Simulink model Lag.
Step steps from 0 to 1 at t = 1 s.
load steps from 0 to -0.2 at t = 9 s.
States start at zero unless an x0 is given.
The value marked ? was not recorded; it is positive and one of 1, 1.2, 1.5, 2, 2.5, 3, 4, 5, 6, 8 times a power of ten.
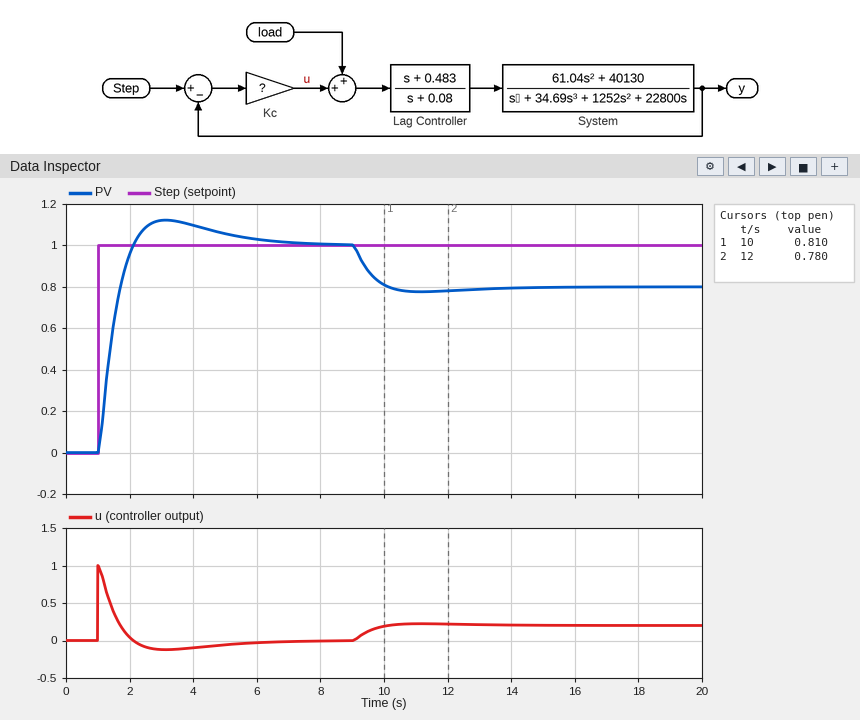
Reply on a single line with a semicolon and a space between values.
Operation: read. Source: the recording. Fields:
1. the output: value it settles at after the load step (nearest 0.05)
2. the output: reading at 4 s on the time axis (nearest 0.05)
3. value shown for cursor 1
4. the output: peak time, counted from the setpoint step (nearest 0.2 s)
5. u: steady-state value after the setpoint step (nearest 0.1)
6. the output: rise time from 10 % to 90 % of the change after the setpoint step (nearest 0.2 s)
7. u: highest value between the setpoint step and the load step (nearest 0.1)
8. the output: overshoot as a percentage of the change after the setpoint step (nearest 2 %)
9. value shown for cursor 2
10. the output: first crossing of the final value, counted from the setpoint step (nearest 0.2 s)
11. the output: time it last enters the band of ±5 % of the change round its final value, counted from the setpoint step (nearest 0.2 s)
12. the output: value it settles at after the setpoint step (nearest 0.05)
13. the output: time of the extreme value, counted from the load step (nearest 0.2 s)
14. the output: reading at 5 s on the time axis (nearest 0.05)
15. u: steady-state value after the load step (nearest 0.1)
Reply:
0.80; 1.10; 0.810; 2.2 s; 0.0; 0.8 s; 1.0; 12 %; 0.780; 1.2 s; 4.2 s; 1.00; 2.2 s; 1.05; 0.2
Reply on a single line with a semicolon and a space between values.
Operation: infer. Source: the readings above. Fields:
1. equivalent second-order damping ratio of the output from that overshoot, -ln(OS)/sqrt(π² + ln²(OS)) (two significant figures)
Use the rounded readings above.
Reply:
0.56
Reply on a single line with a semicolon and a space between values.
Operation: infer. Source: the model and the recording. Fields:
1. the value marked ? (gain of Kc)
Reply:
1
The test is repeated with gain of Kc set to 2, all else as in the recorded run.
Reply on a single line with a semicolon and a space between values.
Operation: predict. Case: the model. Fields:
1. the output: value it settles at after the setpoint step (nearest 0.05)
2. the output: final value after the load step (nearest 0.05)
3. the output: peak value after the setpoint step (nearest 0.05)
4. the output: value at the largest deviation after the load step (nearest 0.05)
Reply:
1.00; 0.90; 1.10; 0.90
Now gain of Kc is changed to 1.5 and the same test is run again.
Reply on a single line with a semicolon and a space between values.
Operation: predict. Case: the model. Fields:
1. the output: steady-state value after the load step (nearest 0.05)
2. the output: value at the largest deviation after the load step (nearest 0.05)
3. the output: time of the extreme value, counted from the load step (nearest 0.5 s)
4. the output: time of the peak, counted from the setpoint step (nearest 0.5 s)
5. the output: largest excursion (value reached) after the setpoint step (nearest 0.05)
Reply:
0.85; 0.85; 1.5 s; 1.5 s; 1.10
